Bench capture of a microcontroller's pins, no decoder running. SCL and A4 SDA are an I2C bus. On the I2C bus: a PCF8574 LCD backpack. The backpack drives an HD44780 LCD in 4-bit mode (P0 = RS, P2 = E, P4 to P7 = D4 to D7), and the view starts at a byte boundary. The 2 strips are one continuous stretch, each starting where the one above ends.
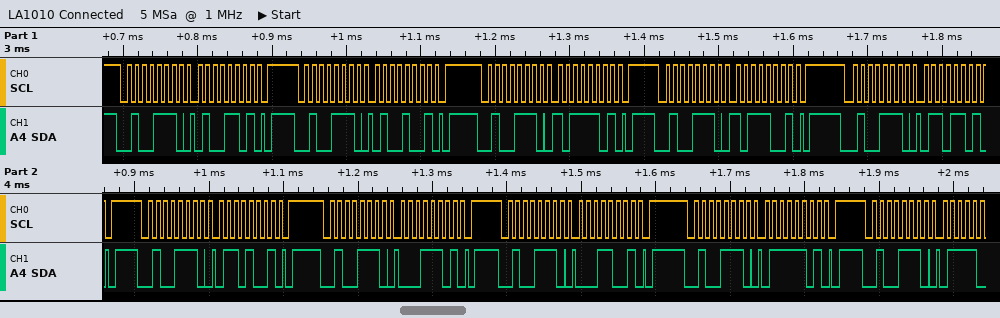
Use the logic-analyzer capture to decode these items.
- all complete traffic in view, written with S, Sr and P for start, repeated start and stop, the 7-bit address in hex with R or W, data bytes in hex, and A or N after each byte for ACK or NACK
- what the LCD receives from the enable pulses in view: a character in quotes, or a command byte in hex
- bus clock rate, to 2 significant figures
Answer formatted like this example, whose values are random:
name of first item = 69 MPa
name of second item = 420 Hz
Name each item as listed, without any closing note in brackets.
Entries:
all complete traffic in view, written with S, Sr and P for start, repeated start and stop, the 7-bit address in hex with R or W, data bytes in hex, and A or N after each byte for ACK or NACK = S 27W A 4D A P S 27W A 49 A P S 27W A BD A P S 27W A B9 A P S 27W A 6D A P S 27W A 69 A P S 27W A 1D A P S 27W A 19 A P S 27W A 7D A P S 27W A
what the LCD receives from the enable pulses in view: a character in quotes, or a command byte in hex = 'K' 'a'
bus clock rate, to 2 significant figures = 100 kHz
